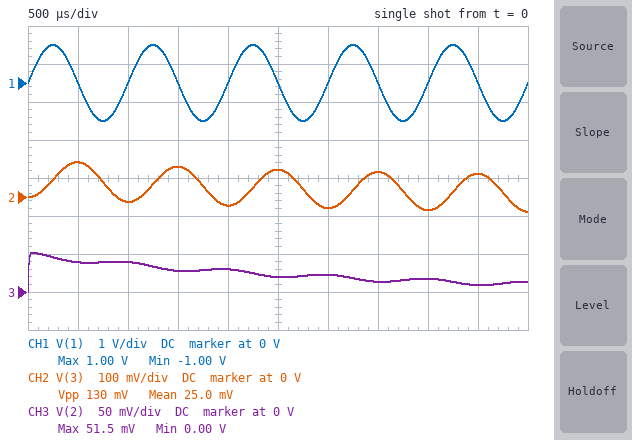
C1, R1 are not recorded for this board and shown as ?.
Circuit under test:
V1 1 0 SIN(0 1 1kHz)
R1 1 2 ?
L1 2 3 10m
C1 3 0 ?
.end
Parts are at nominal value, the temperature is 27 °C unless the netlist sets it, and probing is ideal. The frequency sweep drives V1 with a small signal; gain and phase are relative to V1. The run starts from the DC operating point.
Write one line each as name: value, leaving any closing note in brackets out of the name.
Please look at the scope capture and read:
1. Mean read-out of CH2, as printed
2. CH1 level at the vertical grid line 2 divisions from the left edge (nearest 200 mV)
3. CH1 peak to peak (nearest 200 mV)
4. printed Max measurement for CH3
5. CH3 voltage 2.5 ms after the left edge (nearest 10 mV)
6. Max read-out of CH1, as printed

Mean read-out of CH2, as printed: 25.0 mV
CH1 level at the vertical grid line 2 divisions from the left edge: 0 V
CH1 peak to peak: 2.0 V
printed Max measurement for CH3: 51.5 mV
CH3 voltage 2.5 ms after the left edge: 20 mV
Max read-out of CH1, as printed: 1.00 V
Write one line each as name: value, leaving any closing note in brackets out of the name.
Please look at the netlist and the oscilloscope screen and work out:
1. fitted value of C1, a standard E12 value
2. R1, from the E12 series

fitted value of C1, a standard E12 value: 2.7 µF
R1, from the E12 series: 1.2 kΩ
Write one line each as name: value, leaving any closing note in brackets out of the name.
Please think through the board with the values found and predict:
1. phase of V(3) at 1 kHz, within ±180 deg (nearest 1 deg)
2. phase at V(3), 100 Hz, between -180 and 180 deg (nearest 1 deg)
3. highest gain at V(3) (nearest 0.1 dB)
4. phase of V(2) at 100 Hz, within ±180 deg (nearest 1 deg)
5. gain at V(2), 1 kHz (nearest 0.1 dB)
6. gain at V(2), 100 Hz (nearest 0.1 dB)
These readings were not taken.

phase of V(3) at 1 kHz, within ±180 deg: -90 deg
phase at V(3), 100 Hz, between -180 and 180 deg: -64 deg
highest gain at V(3): 0 dB
phase of V(2) at 100 Hz, within ±180 deg: -64 deg
gain at V(2), 1 kHz: -49.8 dB
gain at V(2), 100 Hz: -7.2 dB
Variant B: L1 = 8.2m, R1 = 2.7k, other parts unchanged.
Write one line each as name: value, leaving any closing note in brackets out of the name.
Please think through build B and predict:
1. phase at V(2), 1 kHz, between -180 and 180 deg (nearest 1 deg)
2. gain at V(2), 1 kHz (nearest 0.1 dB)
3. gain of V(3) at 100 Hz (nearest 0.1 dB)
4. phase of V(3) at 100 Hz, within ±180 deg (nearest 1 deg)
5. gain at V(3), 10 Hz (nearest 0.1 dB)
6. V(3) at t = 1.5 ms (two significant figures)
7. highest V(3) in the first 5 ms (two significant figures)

phase at V(2), 1 kHz, between -180 and 180 deg: -90 deg
gain at V(2), 1 kHz: -51.2 dB
gain of V(3) at 100 Hz: -13.4 dB
phase of V(3) at 100 Hz, within ±180 deg: -78 deg
gain at V(3), 10 Hz: -0.8 dB
V(3) at t = 1.5 ms: 40 mV
highest V(3) in the first 5 ms: 42 mV
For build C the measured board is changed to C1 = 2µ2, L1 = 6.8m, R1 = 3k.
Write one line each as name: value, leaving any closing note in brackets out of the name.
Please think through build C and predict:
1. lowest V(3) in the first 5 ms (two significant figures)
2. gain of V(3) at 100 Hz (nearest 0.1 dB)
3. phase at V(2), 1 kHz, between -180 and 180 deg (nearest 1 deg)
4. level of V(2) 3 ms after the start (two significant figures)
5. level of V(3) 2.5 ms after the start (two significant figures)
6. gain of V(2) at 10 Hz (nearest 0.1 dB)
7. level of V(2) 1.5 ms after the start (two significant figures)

lowest V(3) in the first 5 ms: -13 mV
gain of V(3) at 100 Hz: -12.6 dB
phase at V(2), 1 kHz, between -180 and 180 deg: -89 deg
level of V(2) 3 ms after the start: 5.4 mV
level of V(3) 2.5 ms after the start: 41 mV
gain of V(2) at 10 Hz: -0.7 dB
level of V(2) 1.5 ms after the start: 29 mV
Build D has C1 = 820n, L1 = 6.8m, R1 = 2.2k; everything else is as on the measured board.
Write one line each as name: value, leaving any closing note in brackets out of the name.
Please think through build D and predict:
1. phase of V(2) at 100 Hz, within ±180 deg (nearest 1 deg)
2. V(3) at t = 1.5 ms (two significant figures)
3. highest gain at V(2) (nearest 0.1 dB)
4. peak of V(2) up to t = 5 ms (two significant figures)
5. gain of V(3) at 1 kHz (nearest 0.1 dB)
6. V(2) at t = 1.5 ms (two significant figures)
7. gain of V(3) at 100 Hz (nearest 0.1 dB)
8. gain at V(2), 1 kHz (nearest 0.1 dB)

phase of V(2) at 100 Hz, within ±180 deg: -49 deg
V(3) at t = 1.5 ms: 130 mV
highest gain at V(2): 0 dB
peak of V(2) up to t = 5 ms: 140 mV
gain of V(3) at 1 kHz: -21.1 dB
V(2) at t = 1.5 ms: 110 mV
gain of V(3) at 100 Hz: -3.6 dB
gain at V(2), 1 kHz: -23.3 dB
